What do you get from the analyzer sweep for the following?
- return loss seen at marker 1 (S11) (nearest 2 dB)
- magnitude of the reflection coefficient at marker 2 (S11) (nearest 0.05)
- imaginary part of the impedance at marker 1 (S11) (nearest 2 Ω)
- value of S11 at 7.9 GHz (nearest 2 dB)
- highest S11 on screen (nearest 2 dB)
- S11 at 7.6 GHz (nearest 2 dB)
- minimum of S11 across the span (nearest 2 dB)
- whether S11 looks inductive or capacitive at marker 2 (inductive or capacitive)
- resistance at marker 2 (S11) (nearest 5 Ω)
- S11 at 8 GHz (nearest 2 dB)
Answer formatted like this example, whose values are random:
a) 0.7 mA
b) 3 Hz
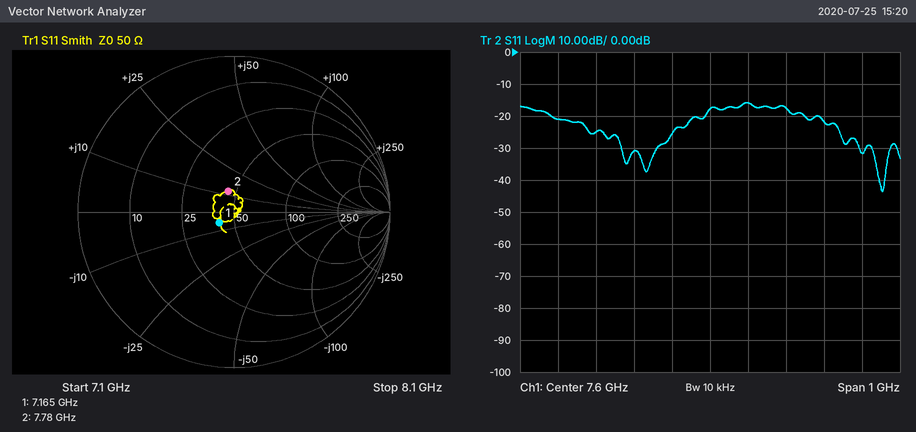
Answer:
a) 18 dB
b) 0.15
c) -6 Ω
d) -22 dB
e) -16 dB
f) -18 dB
g) -44 dB
h) inductive
i) 45 Ω
j) -32 dB
